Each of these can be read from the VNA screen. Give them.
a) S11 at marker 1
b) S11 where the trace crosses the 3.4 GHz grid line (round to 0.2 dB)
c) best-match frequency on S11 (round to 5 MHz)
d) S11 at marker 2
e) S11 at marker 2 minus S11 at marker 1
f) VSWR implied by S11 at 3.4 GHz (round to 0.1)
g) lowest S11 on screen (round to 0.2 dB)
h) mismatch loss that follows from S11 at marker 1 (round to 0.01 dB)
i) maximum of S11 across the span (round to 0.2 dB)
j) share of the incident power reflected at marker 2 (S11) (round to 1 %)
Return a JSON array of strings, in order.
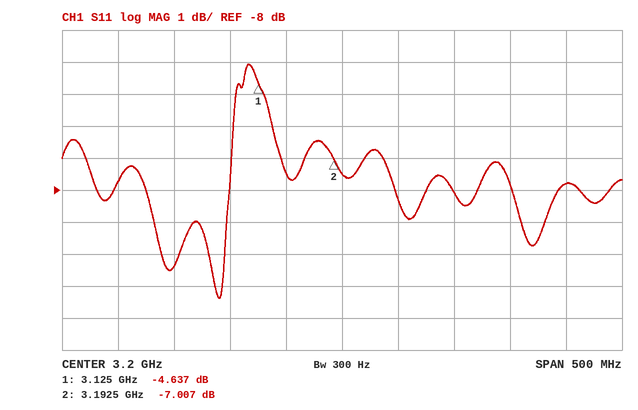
["-4.637 dB", "-7.8 dB", "3.090 GHz", "-7.007 dB", "-2.370 dB", "2.4", "-11.4 dB", "1.83 dB", "-4.0 dB", "20 %"]
